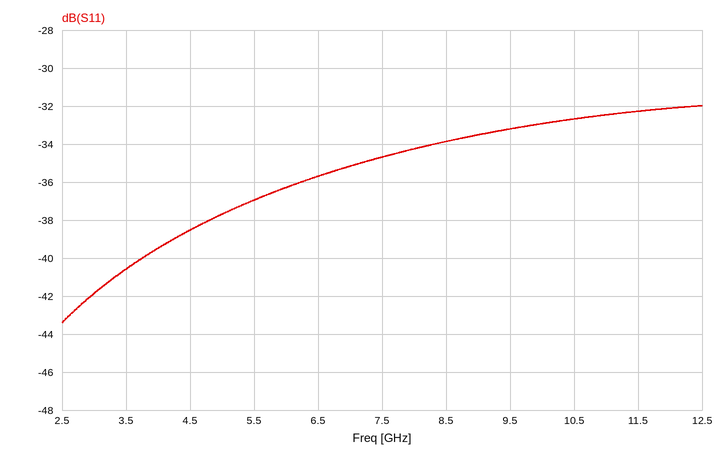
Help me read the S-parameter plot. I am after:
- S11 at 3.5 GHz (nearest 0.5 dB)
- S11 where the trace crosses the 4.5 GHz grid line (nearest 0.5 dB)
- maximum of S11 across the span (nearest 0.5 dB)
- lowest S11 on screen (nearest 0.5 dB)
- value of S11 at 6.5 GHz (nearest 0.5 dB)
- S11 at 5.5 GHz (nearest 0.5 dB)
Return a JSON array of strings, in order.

["-40.5 dB", "-38.5 dB", "-32.0 dB", "-43.5 dB", "-35.5 dB", "-37.0 dB"]
